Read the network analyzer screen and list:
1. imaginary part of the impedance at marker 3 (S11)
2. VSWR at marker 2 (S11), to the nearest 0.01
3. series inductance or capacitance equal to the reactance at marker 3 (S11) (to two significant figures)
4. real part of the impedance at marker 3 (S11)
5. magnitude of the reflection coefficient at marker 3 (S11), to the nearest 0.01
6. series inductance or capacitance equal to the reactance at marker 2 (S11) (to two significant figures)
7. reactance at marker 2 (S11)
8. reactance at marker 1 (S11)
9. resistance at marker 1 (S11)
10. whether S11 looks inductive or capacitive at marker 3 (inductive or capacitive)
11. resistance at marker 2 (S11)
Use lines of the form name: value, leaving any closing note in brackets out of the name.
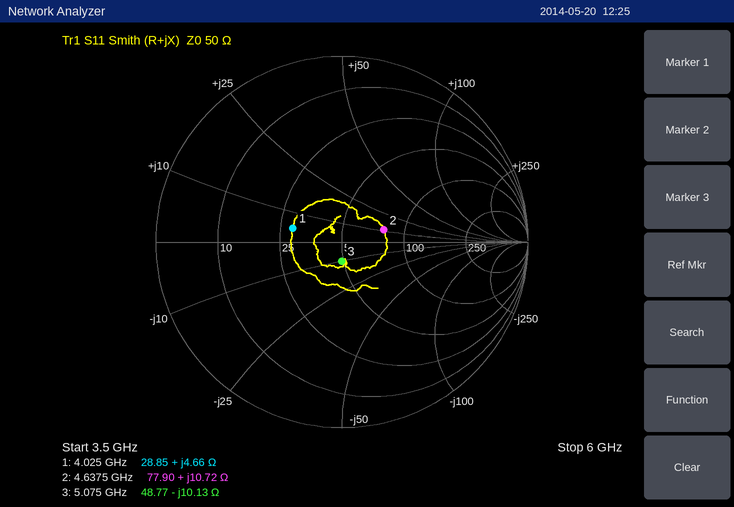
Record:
imaginary part of the impedance at marker 3: -10.13 Ω
VSWR at marker 2 (S11), to the nearest 0.01: 1.61
series inductance or capacitance equal to the reactance at marker 3 (S11): 3.1 pF
real part of the impedance at marker 3: 48.77 Ω
magnitude of the reflection coefficient at marker 3 (S11), to the nearest 0.01: 0.10
series inductance or capacitance equal to the reactance at marker 2 (S11): 370 pH
reactance at marker 2: +10.72 Ω
reactance at marker 1: +4.66 Ω
resistance at marker 1: 28.85 Ω
whether S11 looks inductive or capacitive at marker 3: capacitive
resistance at marker 2: 77.90 Ω
